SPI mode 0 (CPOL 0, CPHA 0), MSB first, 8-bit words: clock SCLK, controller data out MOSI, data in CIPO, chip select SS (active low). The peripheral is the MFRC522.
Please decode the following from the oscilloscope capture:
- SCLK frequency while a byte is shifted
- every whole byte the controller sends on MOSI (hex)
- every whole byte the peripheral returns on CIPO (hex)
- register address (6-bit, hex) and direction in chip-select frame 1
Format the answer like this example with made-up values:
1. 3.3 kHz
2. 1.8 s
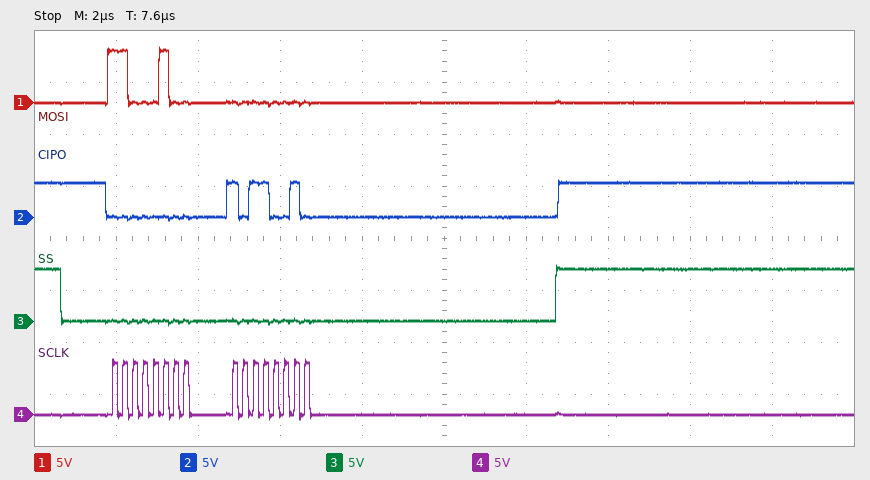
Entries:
1. 4 MHz
2. C4 00
3. 00 B2
4. 0x22 read
